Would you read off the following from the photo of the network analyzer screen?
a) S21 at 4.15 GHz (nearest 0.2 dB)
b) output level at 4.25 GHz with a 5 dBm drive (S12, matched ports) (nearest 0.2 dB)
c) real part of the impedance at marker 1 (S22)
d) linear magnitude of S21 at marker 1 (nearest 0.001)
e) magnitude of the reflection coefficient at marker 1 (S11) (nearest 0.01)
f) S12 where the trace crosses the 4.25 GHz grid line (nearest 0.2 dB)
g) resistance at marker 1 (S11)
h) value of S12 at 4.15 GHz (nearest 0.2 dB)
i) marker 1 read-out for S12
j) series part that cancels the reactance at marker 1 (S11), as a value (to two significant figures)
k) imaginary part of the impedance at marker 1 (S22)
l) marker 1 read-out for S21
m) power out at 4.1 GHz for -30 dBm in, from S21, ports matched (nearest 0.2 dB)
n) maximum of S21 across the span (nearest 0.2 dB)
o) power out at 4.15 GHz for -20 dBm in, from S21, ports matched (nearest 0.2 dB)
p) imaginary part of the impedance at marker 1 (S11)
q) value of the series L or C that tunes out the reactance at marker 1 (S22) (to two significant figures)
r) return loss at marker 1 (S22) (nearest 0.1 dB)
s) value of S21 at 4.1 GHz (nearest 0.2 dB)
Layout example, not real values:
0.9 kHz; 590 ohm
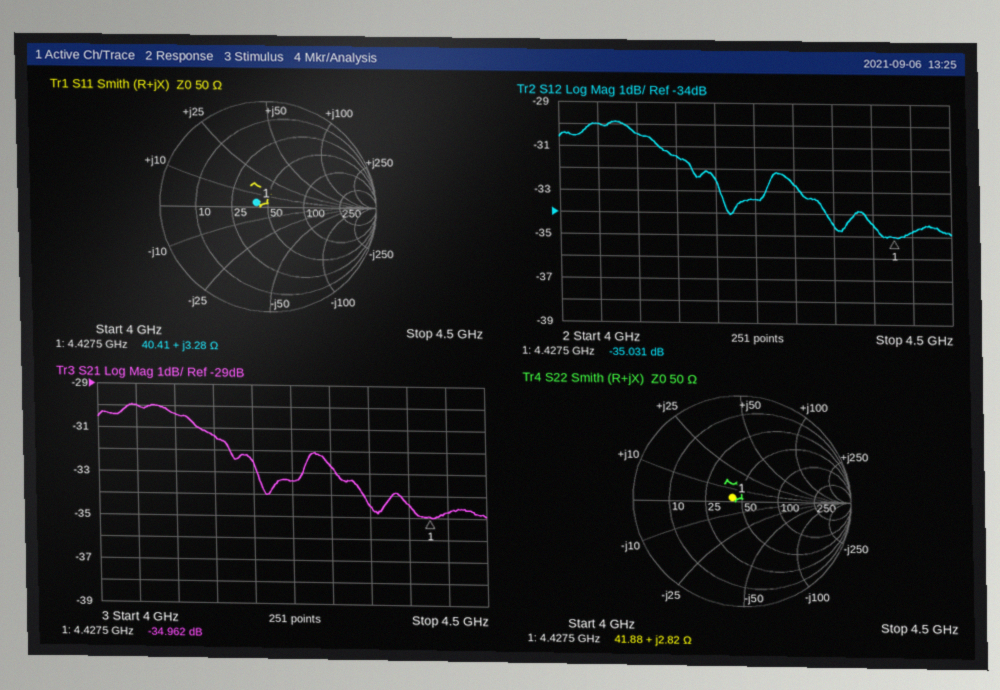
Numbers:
-31.4 dB; -28.4 dBm; 41.88 Ω; 0.018; 0.11; -33.4 dB; 40.41 Ω; -31.4 dB; -35.031 dB; 11 pF; +2.82 Ω; -34.962 dB; -60.4 dBm; -30.0 dB; -51.4 dBm; +3.28 Ω; 13 pF; 20.6 dB; -30.4 dB
